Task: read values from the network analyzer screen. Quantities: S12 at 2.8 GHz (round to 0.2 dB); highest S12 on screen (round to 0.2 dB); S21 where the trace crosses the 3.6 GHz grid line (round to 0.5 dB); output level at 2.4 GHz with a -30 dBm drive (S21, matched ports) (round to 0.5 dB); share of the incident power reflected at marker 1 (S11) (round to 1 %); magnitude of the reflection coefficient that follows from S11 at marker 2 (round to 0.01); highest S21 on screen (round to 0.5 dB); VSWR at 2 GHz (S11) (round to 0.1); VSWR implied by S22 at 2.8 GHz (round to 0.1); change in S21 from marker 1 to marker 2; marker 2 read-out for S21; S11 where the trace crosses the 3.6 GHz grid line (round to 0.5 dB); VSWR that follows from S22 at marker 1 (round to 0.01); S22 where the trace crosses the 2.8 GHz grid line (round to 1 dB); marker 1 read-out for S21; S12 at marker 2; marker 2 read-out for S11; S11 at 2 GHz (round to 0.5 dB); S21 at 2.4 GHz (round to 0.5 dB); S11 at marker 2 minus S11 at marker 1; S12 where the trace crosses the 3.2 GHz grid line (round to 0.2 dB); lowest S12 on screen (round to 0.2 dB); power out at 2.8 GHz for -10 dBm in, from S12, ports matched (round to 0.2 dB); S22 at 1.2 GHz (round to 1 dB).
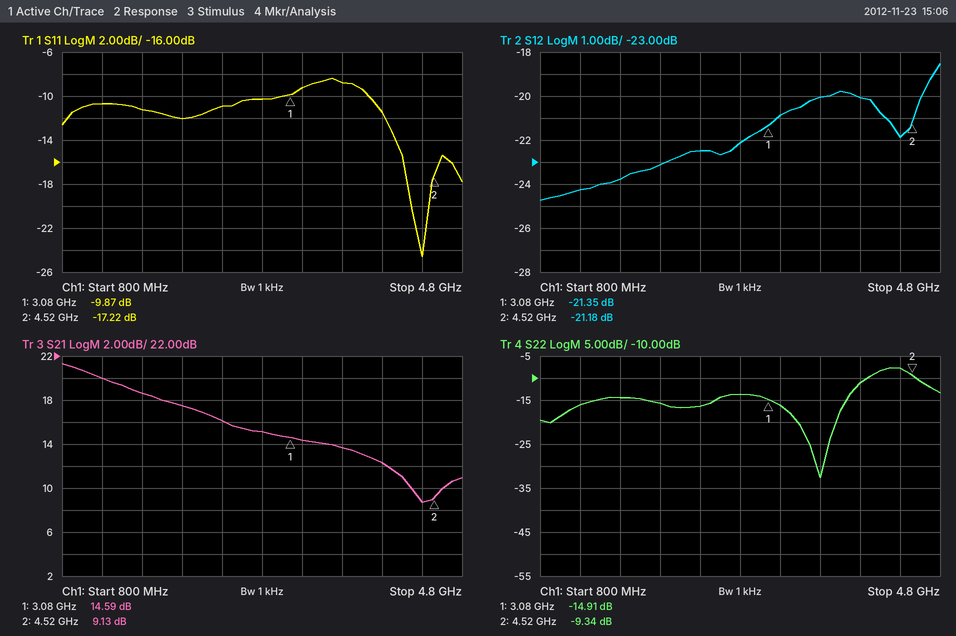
-22.2 dB
-18.6 dB
13.5 dB
-14.0 dBm
10 %
0.14
21.5 dB
1.7
1.5
-5.46 dB
9.13 dB
-9.0 dB
1.44
-14 dB
14.59 dB
-21.18 dB
-17.22 dB
-12.0 dB
16.0 dB
-7.35 dB
-20.8 dB
-24.8 dB
-32.2 dBm
-16 dB
